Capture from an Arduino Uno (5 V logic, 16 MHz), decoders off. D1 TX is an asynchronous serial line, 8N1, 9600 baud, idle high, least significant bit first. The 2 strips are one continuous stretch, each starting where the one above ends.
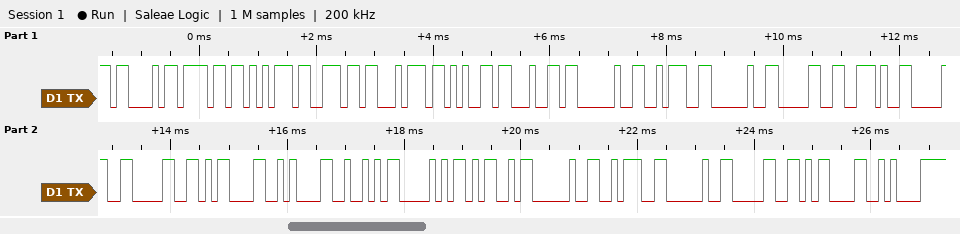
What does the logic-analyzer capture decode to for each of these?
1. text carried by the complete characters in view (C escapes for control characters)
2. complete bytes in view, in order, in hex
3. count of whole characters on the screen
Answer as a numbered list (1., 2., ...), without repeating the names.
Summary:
1. "Counted : 0.00\r\nRPM : 0\r\n"
2. 43 6F 75 6E 74 65 64 20 3A 20 30 2E 30 30 0D 0A 52 50 4D 20 3A 20 30 0D 0A
3. 25
